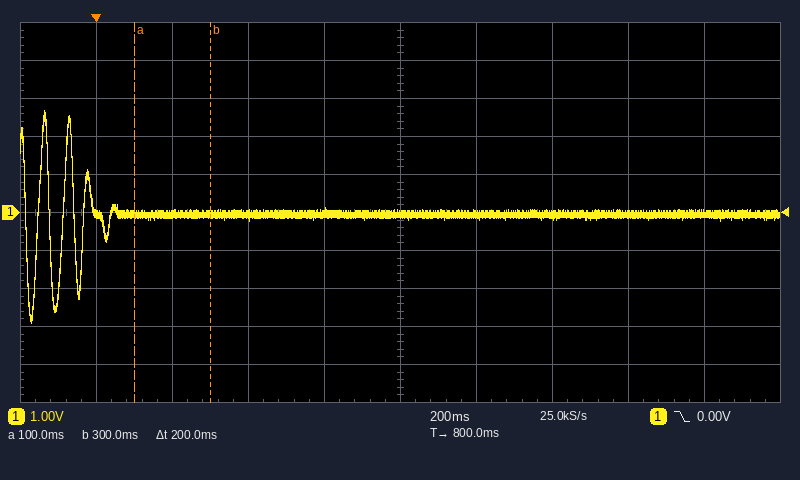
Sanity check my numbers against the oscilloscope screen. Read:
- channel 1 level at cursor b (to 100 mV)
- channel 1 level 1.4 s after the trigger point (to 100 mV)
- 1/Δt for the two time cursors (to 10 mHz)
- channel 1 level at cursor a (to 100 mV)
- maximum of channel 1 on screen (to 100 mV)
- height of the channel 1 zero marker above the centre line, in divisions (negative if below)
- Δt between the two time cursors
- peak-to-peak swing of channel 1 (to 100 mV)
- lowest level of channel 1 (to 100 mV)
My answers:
-100 mV
-100 mV
5.00 Hz
-100 mV
2.7 V
0.0 div
200 ms
5.6 V
-2.9 V
